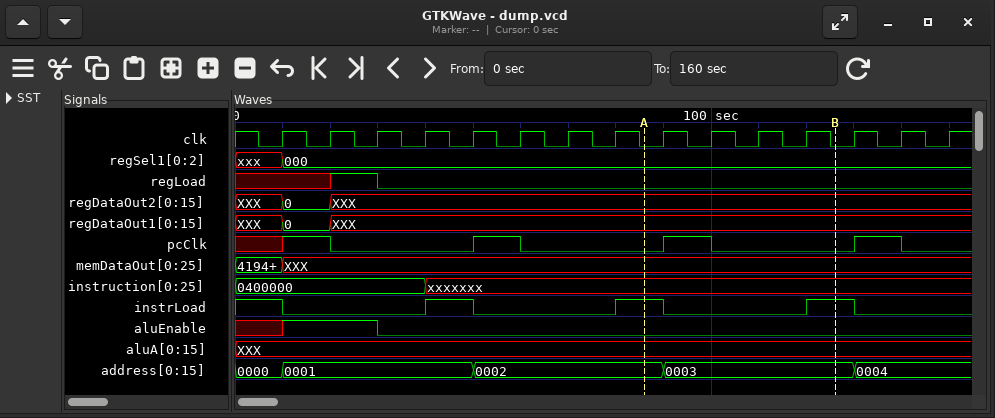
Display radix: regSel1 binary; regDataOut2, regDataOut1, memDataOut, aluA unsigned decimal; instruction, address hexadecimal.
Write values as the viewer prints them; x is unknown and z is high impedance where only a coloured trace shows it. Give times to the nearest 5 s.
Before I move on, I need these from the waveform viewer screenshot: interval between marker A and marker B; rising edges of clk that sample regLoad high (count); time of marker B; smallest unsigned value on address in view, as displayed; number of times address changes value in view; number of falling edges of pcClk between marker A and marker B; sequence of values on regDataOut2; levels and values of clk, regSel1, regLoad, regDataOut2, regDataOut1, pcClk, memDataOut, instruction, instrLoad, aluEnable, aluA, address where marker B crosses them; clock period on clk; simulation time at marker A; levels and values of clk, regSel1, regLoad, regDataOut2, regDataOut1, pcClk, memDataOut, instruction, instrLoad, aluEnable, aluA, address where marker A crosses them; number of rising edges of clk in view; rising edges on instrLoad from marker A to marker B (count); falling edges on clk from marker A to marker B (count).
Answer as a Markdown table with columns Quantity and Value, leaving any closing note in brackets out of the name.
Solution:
| Quantity | Value |
|---|---|
| interval between marker A and marker B | 40 s |
| rising edges of clk that sample regLoad high | 1 |
| time of marker B | 125 s |
| smallest unsigned value on address in view, as displayed | 0000 |
| number of times address changes value in view | 4 |
| number of falling edges of pcClk between marker A and marker B | 1 |
| sequence of values on regDataOut2 | XXX, 0, XXX |
| levels and values of clk, regSel1, regLoad, regDataOut2, regDataOut1, pcClk, memDataOut, instruction, instrLoad, aluEnable, aluA, address where marker B crosses them | clk=0, regSel1=000, regLoad=0, regDataOut2=XXX, regDataOut1=XXX, pcClk=0, memDataOut=XXX, instruction=xxxxxxx, instrLoad=1, aluEnable=0, aluA=XXX, address=0003 |
| clock period on clk | 10 s |
| simulation time at marker A | 85 s |
| levels and values of clk, regSel1, regLoad, regDataOut2, regDataOut1, pcClk, memDataOut, instruction, instrLoad, aluEnable, aluA, address where marker A crosses them | clk=0, regSel1=000, regLoad=0, regDataOut2=XXX, regDataOut1=XXX, pcClk=0, memDataOut=XXX, instruction=xxxxxxx, instrLoad=1, aluEnable=0, aluA=XXX, address=0002 |
| number of rising edges of clk in view | 15 |
| rising edges on instrLoad from marker A to marker B | 1 |
| falling edges on clk from marker A to marker B | 4 |
